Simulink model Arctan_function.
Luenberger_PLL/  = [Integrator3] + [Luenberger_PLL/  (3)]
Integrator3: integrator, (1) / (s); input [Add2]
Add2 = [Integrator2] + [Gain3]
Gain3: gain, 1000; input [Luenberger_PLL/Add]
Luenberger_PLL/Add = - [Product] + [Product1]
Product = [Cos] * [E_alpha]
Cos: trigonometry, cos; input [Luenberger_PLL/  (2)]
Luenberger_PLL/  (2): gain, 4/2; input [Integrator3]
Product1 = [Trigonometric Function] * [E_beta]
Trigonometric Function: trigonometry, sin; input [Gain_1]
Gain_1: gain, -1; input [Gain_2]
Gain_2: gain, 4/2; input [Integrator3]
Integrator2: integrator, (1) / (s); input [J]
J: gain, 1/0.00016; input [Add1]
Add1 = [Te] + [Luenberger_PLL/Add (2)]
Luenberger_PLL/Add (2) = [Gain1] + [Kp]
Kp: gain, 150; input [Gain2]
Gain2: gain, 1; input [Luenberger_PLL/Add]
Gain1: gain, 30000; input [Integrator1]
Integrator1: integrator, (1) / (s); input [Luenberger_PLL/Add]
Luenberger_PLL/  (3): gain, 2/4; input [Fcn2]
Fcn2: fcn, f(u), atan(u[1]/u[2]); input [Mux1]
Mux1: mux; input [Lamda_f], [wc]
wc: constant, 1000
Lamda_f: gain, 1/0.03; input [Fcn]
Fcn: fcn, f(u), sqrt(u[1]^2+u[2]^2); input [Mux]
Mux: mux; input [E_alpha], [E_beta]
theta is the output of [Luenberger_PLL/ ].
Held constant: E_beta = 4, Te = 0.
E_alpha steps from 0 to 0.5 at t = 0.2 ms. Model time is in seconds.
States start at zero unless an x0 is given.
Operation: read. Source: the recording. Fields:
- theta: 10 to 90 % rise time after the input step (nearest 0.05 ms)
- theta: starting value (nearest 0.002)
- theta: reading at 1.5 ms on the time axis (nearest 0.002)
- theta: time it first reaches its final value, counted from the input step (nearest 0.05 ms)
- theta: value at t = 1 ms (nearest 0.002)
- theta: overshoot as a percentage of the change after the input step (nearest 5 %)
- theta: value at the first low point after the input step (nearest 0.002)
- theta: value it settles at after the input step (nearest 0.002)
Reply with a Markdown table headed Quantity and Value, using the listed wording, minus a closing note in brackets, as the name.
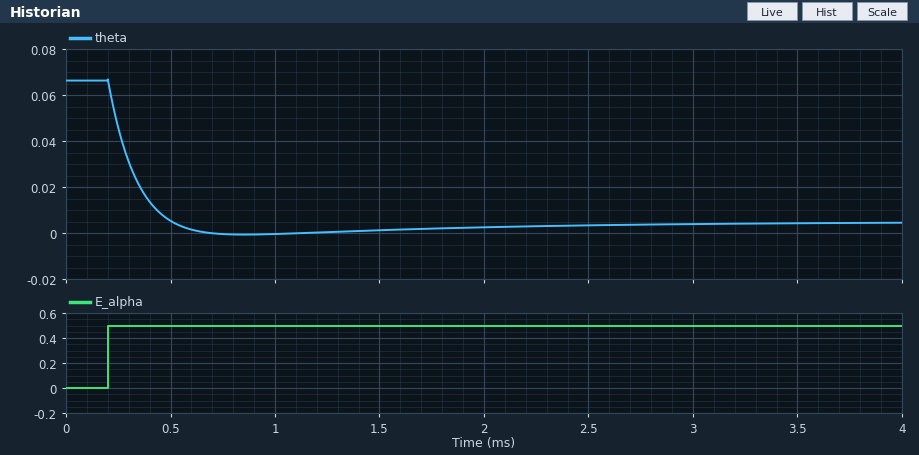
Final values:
| Quantity | Value |
|---|---|
| theta: 10 to 90 % rise time after the input step | 0.20 ms |
| theta: starting value | 0.066 |
| theta: reading at 1.5 ms on the time axis | 0.002 |
| theta: time it first reaches its final value, counted from the input step | 0.30 ms |
| theta: value at t = 1 ms | 0.000 |
| theta: overshoot as a percentage of the change after the input step | 10 % |
| theta: value at the first low point after the input step | 0.000 |
| theta: value it settles at after the input step | 0.004 |
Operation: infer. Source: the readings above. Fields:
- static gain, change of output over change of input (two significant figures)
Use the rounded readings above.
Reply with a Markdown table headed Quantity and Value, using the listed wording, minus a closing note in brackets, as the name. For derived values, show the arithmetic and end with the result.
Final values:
| Quantity | Value |
|---|---|
| static gain, change of output over change of input | (0.004 - 0.066) / (0.5 - 0) = -0.12 |
